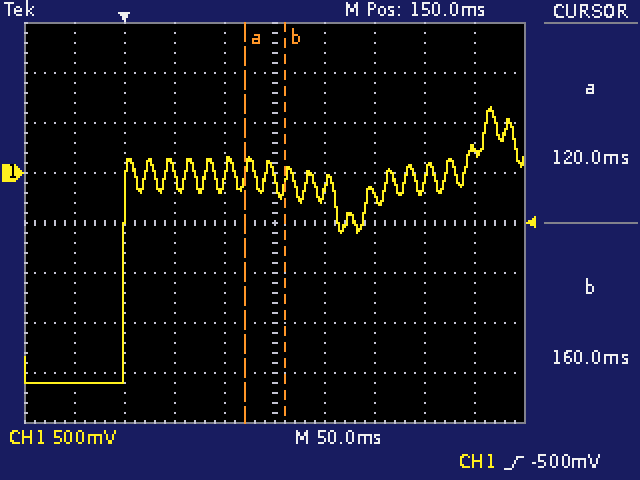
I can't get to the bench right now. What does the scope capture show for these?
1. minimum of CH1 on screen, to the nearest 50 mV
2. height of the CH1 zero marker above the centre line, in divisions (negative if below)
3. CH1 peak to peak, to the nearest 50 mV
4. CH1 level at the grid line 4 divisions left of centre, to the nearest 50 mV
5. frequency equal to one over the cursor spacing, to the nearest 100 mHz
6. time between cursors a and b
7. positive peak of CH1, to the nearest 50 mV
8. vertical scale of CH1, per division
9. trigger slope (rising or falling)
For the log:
-2.10 V
+1.0 div
2.75 V
-2.10 V
25.0 Hz
40 ms
650 mV
500 mV
rising
